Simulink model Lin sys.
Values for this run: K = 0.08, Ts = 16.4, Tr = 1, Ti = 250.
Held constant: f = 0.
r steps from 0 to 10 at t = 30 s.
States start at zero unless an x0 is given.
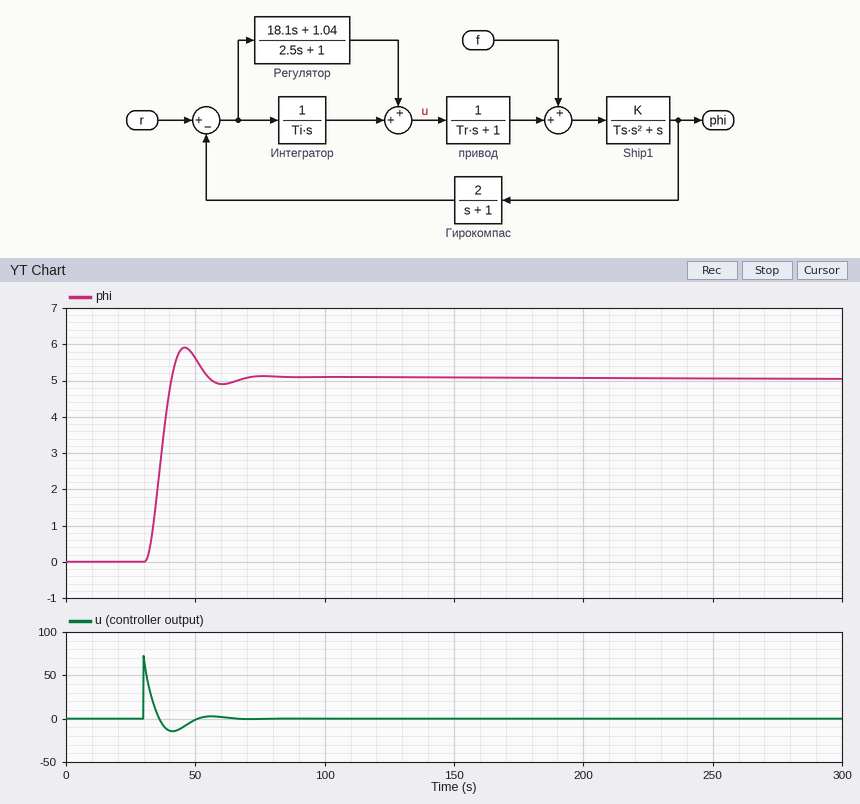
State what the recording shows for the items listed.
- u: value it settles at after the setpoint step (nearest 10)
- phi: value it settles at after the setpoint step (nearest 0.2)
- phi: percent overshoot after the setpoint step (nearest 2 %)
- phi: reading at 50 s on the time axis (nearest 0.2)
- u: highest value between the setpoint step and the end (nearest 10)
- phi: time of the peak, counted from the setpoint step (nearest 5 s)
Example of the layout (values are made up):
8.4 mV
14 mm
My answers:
0
5.0
18 %
5.6
70
15 s
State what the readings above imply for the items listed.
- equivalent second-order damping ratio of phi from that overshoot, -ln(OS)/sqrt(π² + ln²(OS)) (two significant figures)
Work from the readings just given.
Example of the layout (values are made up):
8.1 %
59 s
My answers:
0.48
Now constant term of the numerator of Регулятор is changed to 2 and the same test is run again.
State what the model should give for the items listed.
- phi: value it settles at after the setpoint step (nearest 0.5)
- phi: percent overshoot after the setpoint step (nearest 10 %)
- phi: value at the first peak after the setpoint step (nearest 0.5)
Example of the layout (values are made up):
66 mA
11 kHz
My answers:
5.0
40 %
7.0
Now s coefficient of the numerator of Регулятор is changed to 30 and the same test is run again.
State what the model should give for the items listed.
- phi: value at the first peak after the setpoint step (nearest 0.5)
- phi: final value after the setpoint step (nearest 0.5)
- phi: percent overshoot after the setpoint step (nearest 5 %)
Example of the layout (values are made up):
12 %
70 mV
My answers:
6.5
5.0
30 %
